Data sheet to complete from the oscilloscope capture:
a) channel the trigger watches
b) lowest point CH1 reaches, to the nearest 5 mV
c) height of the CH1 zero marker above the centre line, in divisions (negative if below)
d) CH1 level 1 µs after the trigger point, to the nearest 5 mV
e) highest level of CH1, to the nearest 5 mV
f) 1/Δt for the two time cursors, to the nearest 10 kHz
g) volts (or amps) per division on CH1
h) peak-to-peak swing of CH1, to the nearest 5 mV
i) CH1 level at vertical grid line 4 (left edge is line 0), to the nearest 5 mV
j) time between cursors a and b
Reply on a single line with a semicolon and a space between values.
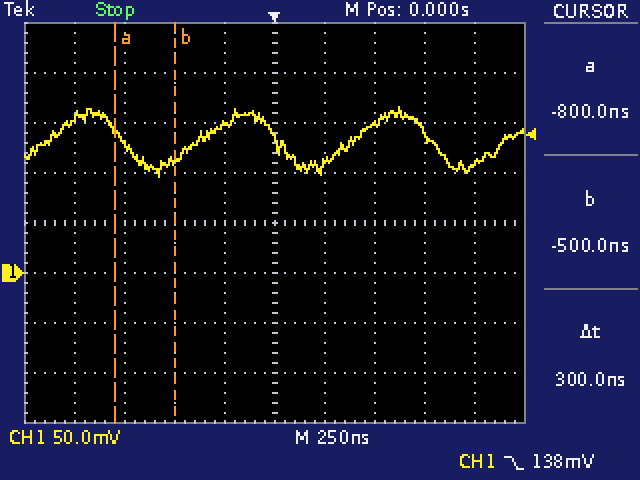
CH1; 95 mV; -1.0 div; 110 mV; 165 mV; 3.33 MHz; 50 mV; 70 mV; 150 mV; 300 ns
